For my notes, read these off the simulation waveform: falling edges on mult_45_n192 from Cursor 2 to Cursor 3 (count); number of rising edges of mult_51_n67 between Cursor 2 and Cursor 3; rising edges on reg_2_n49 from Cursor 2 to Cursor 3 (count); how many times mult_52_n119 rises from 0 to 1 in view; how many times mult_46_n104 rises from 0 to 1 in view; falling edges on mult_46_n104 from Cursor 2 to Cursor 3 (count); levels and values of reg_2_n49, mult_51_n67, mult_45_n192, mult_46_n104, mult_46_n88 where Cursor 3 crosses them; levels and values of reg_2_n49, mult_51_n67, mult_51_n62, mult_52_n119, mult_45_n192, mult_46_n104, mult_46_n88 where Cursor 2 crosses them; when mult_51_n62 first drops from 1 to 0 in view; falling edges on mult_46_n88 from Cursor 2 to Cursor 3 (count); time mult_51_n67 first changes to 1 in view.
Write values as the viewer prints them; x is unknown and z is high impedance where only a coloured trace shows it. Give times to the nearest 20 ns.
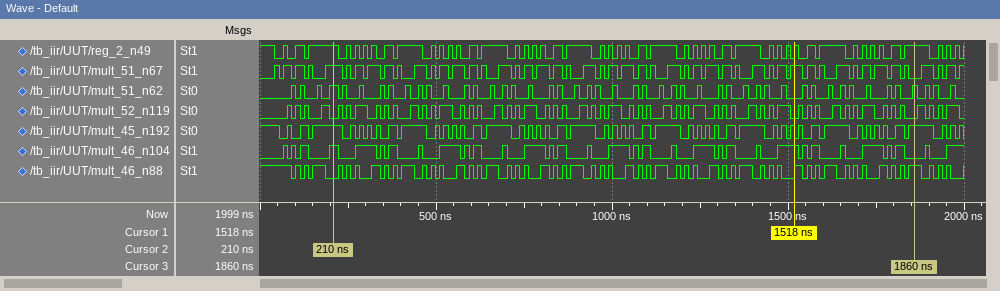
42
41
42
56
33
28
reg_2_n49=1, mult_51_n67=0, mult_45_n192=1, mult_46_n104=0, mult_46_n88=1
reg_2_n49=1, mult_51_n67=1, mult_51_n62=1, mult_52_n119=0, mult_45_n192=1, mult_46_n104=1, mult_46_n88=0
100 ns
48
40 ns
